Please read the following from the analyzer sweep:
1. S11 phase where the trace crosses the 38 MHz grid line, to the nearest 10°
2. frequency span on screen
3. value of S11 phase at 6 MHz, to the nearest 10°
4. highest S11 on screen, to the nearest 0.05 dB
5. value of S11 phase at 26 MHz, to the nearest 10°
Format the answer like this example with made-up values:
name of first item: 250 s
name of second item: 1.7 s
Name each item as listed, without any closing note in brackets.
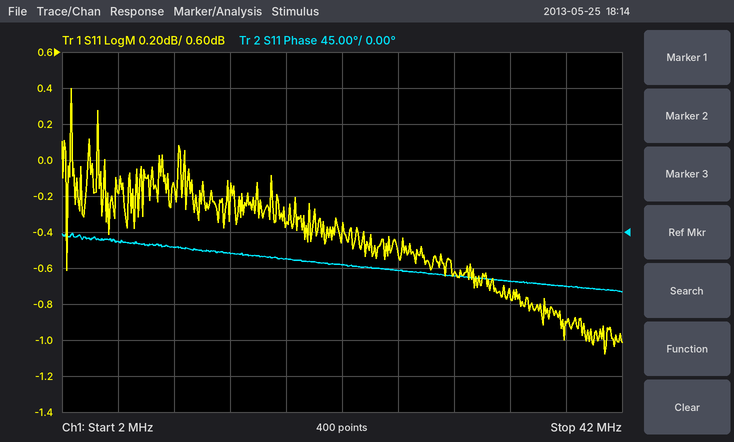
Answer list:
S11 phase where the trace crosses the 38 MHz grid line, to the nearest 10°: -70°
frequency span on screen: 40 MHz
value of S11 phase at 6 MHz, to the nearest 10°: -10°
highest S11 on screen, to the nearest 0.05 dB: 0.40 dB
value of S11 phase at 26 MHz, to the nearest 10°: -50°
